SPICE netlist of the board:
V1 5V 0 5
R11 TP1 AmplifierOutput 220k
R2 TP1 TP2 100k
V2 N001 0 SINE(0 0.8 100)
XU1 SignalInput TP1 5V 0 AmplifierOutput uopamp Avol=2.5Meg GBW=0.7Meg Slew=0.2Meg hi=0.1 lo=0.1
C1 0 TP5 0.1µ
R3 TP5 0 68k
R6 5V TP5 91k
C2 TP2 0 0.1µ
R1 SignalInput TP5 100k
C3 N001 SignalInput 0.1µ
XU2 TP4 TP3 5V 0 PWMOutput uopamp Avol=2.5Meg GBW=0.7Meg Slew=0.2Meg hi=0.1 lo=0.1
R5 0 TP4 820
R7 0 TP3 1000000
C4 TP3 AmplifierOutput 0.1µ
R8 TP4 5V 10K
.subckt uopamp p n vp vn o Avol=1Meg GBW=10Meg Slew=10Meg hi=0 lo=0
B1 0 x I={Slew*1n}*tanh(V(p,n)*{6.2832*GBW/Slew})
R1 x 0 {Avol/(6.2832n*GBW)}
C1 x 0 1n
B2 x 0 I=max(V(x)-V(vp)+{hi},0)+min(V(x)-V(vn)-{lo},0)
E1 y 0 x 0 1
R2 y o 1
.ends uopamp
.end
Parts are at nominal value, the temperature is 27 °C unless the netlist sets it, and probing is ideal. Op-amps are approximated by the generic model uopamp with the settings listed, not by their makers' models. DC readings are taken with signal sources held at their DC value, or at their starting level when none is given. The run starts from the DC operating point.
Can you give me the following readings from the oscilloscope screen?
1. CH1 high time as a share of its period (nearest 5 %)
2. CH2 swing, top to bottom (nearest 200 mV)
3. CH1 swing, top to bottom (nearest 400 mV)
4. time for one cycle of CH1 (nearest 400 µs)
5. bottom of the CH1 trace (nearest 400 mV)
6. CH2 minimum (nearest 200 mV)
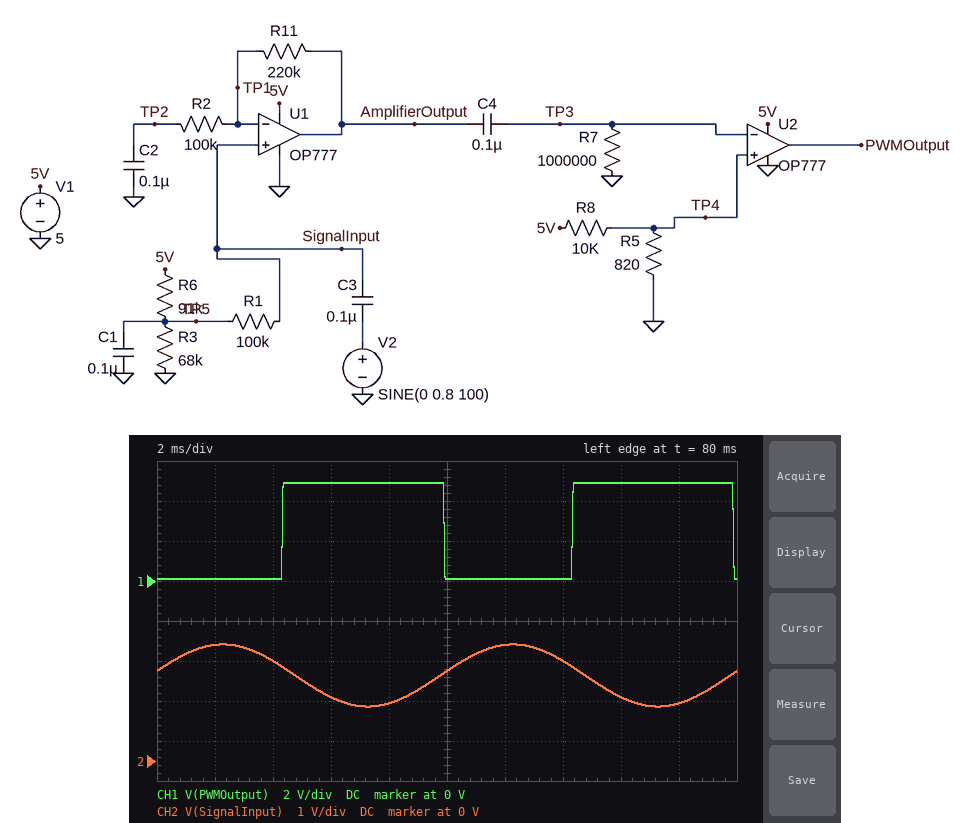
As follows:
55 %
1.6 V
4.8 V
10.0 ms
0 V
1.4 V
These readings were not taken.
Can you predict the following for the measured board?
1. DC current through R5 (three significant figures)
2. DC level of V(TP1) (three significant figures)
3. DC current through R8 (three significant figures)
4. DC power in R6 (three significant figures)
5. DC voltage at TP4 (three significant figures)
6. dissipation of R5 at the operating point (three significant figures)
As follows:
462 µA
2.14 V
462 µA
90.0 µW
379 mV
175 µW
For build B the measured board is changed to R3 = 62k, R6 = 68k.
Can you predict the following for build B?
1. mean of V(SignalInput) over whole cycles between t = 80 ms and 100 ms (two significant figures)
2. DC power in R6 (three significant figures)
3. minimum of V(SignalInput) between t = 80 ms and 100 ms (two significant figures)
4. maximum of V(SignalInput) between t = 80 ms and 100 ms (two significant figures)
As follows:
2.4 V
101 µW
1.6 V
3.2 V
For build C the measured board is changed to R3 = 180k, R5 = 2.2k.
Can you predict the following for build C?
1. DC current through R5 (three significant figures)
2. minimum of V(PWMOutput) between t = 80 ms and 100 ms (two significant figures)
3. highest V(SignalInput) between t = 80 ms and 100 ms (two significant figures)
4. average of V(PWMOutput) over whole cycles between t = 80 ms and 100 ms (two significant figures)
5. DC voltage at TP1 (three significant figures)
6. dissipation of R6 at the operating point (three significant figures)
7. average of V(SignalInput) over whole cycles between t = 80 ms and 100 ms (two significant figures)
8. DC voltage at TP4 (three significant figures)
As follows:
410 µA
100 mV
4.1 V
3.0 V
3.32 V
31.0 µW
3.3 V
902 mV
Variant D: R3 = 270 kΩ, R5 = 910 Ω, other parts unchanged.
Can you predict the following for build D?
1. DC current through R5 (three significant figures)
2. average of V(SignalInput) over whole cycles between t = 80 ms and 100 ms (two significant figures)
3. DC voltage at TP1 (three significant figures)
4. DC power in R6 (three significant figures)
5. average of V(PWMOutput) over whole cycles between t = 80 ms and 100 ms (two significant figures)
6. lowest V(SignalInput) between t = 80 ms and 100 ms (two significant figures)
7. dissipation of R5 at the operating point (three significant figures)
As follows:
458 µA
3.7 V
3.74 V
17.5 µW
2.5 V
3.0 V
191 µW
